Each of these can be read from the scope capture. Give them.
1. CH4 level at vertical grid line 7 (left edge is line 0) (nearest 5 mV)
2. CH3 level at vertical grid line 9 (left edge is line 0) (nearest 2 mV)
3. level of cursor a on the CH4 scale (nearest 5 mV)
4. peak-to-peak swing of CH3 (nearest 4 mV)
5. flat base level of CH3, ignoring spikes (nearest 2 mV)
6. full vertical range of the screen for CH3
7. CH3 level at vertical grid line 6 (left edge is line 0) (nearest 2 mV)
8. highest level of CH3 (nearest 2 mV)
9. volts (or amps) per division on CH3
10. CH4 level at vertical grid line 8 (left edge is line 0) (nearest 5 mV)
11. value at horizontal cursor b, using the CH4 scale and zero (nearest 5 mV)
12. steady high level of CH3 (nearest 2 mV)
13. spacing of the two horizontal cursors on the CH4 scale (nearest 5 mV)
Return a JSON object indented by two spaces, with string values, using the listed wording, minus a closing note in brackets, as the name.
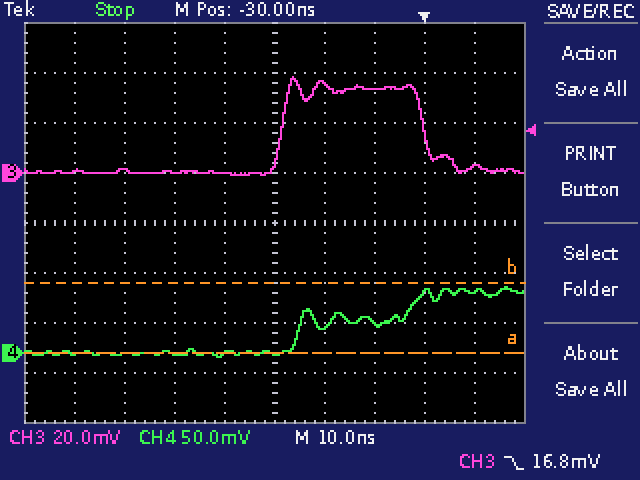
{
  "CH4 level at vertical grid line 7 (left edge is line 0)": "30 mV",
  "CH3 level at vertical grid line 9 (left edge is line 0)": "2 mV",
  "level of cursor a on the CH4 scale": "0 mV",
  "peak-to-peak swing of CH3": "40 mV",
  "flat base level of CH3, ignoring spikes": "0 mV",
  "full vertical range of the screen for CH3": "160 mV",
  "CH3 level at vertical grid line 6 (left edge is line 0)": "36 mV",
  "highest level of CH3": "38 mV",
  "volts (or amps) per division on CH3": "20 mV",
  "CH4 level at vertical grid line 8 (left edge is line 0)": "60 mV",
  "value at horizontal cursor b, using the CH4 scale and zero": "70 mV",
  "steady high level of CH3": "34 mV",
  "spacing of the two horizontal cursors on the CH4 scale": "70 mV"
}
